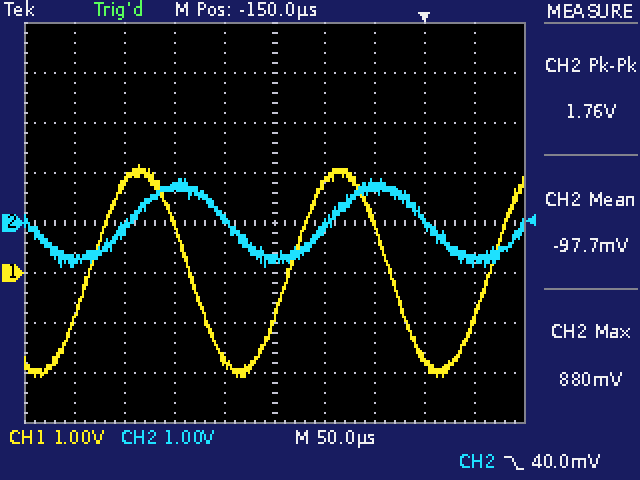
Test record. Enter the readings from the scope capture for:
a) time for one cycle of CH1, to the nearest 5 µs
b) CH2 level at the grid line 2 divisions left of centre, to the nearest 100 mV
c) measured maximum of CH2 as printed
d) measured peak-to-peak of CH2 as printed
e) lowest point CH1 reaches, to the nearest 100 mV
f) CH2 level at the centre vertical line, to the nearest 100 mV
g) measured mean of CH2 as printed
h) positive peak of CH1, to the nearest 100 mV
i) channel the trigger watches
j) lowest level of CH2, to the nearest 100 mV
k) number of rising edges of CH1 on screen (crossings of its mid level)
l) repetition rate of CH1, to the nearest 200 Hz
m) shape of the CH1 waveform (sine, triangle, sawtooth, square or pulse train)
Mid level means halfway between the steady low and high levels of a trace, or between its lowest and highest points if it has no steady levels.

200 µs
700 mV
880 mV
1.76 V
-2.1 V
-700 mV
-97.7 mV
2.2 V
CH2
-900 mV
3
5.0 kHz
sine
